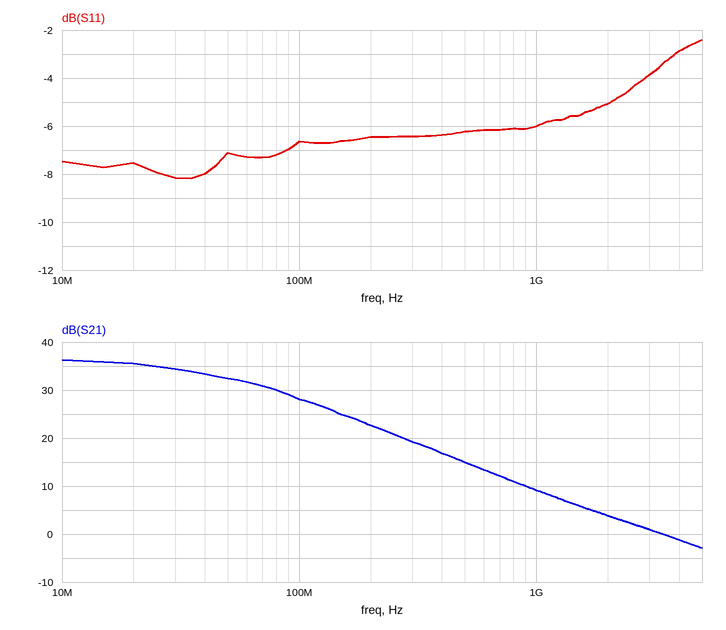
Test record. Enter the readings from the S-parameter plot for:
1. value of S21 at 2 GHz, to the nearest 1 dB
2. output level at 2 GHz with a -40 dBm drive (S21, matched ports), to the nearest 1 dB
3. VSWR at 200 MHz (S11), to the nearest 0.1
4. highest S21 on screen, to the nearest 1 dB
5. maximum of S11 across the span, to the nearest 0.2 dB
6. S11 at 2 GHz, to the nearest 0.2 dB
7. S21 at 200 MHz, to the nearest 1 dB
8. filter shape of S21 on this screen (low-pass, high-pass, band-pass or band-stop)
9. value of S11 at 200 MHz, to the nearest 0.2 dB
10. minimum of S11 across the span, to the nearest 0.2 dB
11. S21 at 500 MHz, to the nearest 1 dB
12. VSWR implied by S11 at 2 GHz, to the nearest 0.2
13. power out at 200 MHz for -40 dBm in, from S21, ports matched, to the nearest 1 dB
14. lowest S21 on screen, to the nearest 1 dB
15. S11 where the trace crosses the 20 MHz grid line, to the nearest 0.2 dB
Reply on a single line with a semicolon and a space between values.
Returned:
4 dB; -36 dBm; 2.8; 36 dB; -2.4 dB; -5.0 dB; 23 dB; low-pass; -6.4 dB; -8.2 dB; 15 dB; 3.6; -17 dBm; -3 dB; -7.6 dB
